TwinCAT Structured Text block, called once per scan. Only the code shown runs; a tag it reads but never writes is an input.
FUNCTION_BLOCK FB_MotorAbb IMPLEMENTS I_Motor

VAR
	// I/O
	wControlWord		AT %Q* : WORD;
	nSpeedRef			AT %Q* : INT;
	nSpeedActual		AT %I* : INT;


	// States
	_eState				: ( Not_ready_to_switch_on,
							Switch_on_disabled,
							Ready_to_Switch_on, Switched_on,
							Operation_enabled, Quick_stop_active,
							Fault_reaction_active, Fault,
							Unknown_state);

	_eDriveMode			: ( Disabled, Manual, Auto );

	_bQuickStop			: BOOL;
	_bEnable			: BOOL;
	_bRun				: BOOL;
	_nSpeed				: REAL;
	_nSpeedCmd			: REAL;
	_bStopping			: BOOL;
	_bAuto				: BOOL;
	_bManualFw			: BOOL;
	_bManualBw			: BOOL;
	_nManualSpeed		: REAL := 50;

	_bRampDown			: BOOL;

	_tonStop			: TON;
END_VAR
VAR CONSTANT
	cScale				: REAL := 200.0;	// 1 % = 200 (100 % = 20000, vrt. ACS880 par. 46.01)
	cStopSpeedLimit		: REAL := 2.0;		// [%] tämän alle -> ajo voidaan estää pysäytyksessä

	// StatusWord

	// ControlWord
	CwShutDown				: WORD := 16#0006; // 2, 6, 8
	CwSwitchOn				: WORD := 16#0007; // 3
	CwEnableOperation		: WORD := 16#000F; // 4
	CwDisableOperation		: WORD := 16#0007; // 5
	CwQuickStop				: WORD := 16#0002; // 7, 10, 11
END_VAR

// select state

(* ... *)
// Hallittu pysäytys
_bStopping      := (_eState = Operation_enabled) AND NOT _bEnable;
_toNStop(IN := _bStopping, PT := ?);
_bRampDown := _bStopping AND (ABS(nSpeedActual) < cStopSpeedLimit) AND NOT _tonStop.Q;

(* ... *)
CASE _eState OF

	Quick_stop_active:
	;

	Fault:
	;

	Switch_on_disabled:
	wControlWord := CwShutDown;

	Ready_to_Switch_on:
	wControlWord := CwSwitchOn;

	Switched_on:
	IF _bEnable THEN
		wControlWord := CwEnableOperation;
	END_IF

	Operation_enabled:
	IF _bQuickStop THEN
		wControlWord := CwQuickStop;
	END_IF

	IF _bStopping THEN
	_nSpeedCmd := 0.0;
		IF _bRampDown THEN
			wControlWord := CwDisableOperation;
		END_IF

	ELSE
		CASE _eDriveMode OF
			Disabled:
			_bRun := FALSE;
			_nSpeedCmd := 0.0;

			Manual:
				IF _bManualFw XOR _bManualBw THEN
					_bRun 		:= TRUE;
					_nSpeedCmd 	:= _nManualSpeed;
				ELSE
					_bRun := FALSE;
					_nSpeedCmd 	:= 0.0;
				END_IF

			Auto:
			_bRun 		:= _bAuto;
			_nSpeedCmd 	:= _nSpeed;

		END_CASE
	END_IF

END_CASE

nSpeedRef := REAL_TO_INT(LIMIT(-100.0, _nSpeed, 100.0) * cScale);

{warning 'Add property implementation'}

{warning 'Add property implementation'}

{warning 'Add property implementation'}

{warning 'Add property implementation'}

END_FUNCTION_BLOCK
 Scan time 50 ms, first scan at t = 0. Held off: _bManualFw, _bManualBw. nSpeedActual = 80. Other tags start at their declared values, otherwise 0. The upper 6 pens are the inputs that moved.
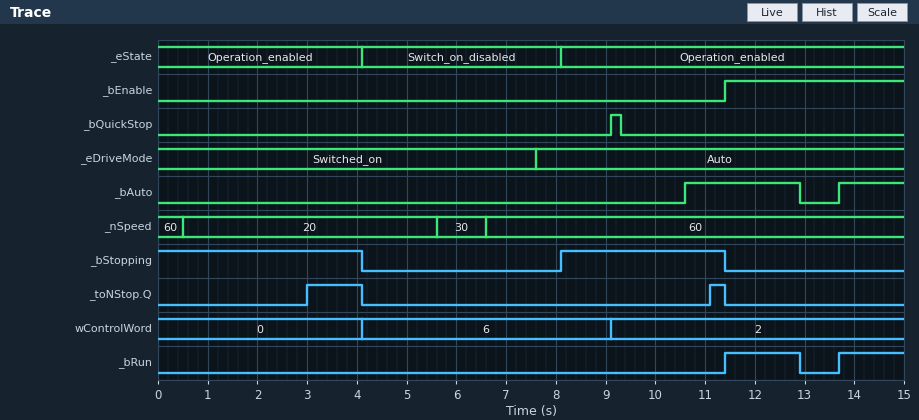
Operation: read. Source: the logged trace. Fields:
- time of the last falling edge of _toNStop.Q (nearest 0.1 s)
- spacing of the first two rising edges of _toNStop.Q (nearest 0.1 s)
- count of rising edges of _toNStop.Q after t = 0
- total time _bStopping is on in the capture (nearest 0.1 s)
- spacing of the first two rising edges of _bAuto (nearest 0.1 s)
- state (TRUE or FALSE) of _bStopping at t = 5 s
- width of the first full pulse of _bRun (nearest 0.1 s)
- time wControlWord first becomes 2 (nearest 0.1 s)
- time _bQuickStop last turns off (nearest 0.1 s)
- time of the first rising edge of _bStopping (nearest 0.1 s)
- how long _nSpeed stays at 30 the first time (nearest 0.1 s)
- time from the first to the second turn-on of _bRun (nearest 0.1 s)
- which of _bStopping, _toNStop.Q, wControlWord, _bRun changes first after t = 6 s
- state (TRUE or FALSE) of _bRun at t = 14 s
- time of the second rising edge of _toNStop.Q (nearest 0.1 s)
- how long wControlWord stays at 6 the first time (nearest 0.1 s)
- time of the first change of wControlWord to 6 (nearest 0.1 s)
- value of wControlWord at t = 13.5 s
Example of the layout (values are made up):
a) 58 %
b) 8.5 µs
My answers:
a) 11.4 s
b) 8.1 s
c) 2
d) 7.4 s
e) 3.1 s
f) FALSE
g) 1.5 s
h) 9.1 s
i) 9.3 s
j) 8.1 s
k) 1.0 s
l) 2.3 s
m) _bStopping
n) TRUE
o) 11.1 s
p) 5.0 s
q) 4.1 s
r) 2
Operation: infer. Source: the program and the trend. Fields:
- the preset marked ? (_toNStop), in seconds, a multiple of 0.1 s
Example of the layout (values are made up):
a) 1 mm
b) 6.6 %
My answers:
a) 3.0 s
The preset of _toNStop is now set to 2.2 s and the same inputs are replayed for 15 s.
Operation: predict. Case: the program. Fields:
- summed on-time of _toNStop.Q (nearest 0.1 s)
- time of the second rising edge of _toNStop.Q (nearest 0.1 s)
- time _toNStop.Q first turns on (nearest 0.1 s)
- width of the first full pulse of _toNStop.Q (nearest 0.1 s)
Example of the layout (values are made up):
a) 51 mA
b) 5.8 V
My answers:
a) 3.0 s
b) 10.3 s
c) 2.2 s
d) 1.9 s
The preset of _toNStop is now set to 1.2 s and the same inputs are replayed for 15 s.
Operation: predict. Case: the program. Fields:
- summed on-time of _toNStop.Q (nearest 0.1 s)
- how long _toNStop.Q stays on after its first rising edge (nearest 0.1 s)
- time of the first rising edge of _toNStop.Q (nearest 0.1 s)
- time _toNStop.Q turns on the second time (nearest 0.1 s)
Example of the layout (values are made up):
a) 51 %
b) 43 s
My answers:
a) 5.0 s
b) 2.9 s
c) 1.2 s
d) 9.3 s
